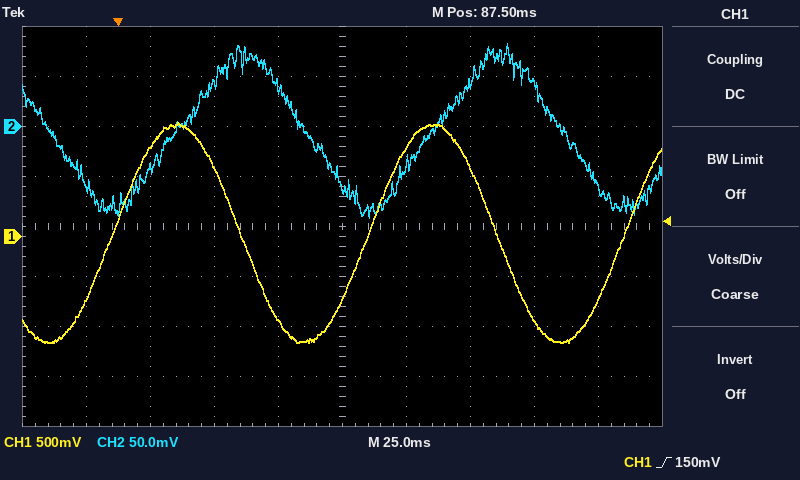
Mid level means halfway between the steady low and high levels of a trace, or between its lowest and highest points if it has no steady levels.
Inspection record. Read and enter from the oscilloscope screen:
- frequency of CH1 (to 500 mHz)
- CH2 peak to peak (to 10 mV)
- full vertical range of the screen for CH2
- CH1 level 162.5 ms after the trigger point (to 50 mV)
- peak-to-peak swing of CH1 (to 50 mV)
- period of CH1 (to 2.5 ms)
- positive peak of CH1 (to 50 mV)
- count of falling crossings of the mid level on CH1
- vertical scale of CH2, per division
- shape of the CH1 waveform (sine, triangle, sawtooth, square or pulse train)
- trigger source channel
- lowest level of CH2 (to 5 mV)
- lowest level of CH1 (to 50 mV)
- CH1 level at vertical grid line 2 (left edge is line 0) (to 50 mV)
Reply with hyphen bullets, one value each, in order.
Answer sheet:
- 10.0 Hz
- 170 mV
- 400 mV
- -850 mV
- 2.20 V
- 100.0 ms
- 1.15 V
- 2
- 50 mV
- sine
- CH1
- -90 mV
- -1.05 V
- 900 mV
